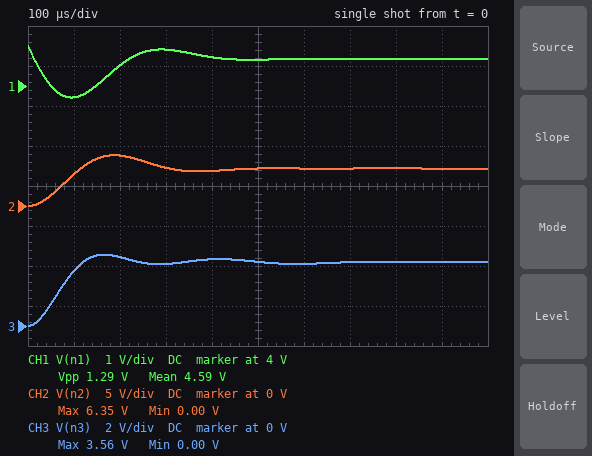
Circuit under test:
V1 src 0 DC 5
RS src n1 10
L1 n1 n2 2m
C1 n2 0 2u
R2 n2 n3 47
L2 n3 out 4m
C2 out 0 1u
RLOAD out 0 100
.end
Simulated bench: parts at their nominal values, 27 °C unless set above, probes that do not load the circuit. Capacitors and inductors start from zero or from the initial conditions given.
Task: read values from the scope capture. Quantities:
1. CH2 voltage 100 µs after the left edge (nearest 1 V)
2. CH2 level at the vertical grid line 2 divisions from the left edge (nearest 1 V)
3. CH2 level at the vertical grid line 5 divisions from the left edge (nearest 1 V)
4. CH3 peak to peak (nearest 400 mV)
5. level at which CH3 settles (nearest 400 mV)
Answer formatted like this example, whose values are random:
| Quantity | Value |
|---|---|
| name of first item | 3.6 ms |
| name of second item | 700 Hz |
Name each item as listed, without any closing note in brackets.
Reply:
| Quantity | Value |
|---|---|
| CH2 voltage 100 µs after the left edge | 4 V |
| CH2 level at the vertical grid line 2 divisions from the left edge | 6 V |
| CH2 level at the vertical grid line 5 divisions from the left edge | 5 V |
| CH3 peak to peak | 3.6 V |
| level at which CH3 settles | 3.2 V |
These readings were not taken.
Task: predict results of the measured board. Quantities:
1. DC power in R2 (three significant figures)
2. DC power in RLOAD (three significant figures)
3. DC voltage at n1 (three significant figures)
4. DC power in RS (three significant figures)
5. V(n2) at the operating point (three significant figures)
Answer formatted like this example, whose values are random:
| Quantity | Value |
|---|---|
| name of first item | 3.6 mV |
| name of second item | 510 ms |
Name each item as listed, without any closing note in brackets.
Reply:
| Quantity | Value |
|---|---|
| DC power in R2 | 47.7 mW |
| DC power in RLOAD | 101 mW |
| DC voltage at n1 | 4.68 V |
| DC power in RS | 10.1 mW |
| V(n2) at the operating point | 4.68 V |
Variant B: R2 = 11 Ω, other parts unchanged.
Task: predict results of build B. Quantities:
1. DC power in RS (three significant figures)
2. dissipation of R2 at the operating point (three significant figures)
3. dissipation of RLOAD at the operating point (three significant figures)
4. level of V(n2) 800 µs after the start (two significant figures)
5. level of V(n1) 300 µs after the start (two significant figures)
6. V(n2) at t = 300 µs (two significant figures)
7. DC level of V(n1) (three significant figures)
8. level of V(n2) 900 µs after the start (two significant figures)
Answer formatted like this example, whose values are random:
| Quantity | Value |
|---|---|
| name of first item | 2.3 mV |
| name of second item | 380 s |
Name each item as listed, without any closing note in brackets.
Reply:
| Quantity | Value |
|---|---|
| DC power in RS | 17.1 mW |
| dissipation of R2 at the operating point | 18.8 mW |
| dissipation of RLOAD at the operating point | 171 mW |
| level of V(n2) 800 µs after the start | 4.6 V |
| level of V(n1) 300 µs after the start | 4.6 V |
| V(n2) at t = 300 µs | 4.4 V |
| DC level of V(n1) | 4.59 V |
| level of V(n2) 900 µs after the start | 4.5 V |
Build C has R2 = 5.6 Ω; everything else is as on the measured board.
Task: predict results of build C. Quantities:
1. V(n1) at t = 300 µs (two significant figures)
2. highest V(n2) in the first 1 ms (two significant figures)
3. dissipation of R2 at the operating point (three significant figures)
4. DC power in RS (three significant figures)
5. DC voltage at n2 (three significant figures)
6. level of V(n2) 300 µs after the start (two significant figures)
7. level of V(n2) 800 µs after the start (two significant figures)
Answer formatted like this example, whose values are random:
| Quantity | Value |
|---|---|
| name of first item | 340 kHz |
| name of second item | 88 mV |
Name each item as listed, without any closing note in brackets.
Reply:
| Quantity | Value |
|---|---|
| V(n1) at t = 300 µs | 4.5 V |
| highest V(n2) in the first 1 ms | 5.8 V |
| dissipation of R2 at the operating point | 10.5 mW |
| DC power in RS | 18.7 mW |
| DC voltage at n2 | 4.57 V |
| level of V(n2) 300 µs after the start | 4.3 V |
| level of V(n2) 800 µs after the start | 4.6 V |
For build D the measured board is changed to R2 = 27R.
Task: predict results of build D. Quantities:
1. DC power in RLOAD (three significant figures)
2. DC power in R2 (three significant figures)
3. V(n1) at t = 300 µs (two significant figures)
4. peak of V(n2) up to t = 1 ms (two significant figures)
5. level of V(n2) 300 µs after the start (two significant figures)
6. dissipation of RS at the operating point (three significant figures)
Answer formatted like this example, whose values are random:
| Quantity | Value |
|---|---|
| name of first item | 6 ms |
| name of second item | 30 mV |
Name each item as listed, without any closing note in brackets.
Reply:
| Quantity | Value |
|---|---|
| DC power in RLOAD | 133 mW |
| DC power in R2 | 36.0 mW |
| V(n1) at t = 300 µs | 4.8 V |
| peak of V(n2) up to t = 1 ms | 6.1 V |
| level of V(n2) 300 µs after the start | 4.6 V |
| dissipation of RS at the operating point | 13.3 mW |
